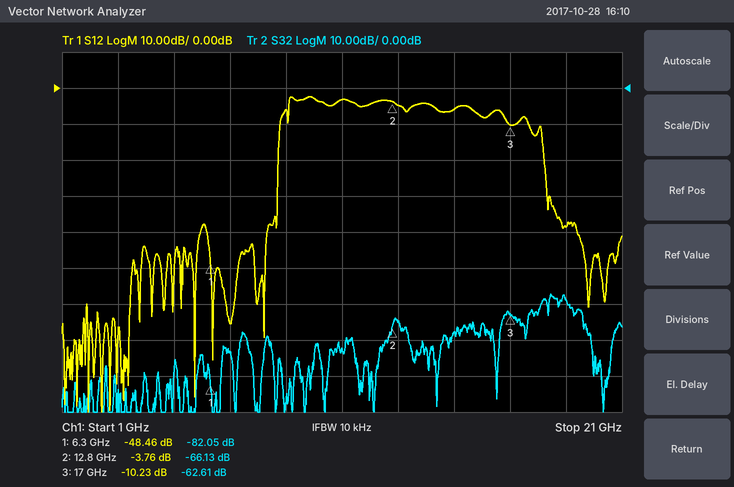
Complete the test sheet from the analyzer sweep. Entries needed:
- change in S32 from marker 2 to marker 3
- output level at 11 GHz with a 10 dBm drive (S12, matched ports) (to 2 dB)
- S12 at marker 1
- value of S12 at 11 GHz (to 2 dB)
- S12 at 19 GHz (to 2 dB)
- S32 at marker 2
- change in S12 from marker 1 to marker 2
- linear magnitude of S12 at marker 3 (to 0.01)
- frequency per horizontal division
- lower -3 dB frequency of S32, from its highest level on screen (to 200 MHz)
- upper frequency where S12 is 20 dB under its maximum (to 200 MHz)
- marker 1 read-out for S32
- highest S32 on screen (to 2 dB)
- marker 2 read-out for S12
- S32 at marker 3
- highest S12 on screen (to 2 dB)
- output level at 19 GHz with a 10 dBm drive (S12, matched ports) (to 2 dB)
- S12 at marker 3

3.52 dB
6 dBm
-48.46 dB
-4 dB
-38 dB
-66.13 dB
44.70 dB
0.31
2 GHz
18.4 GHz
18.2 GHz
-82.05 dB
-58 dB
-3.76 dB
-62.61 dB
-2 dB
-28 dBm
-10.23 dB
